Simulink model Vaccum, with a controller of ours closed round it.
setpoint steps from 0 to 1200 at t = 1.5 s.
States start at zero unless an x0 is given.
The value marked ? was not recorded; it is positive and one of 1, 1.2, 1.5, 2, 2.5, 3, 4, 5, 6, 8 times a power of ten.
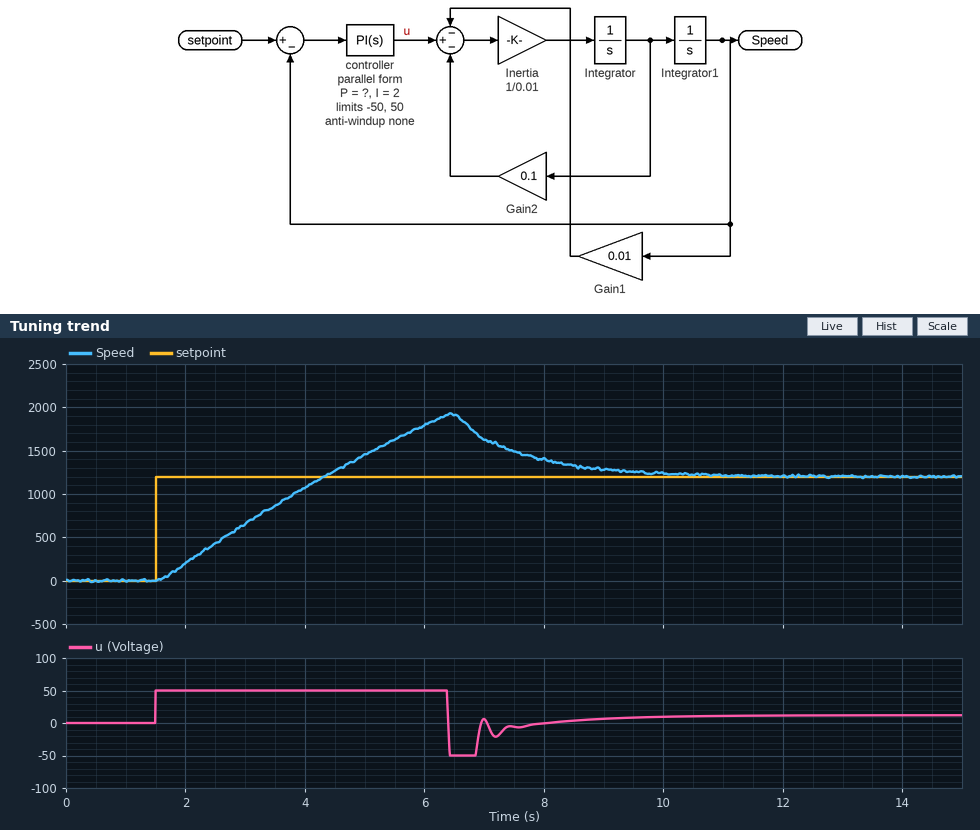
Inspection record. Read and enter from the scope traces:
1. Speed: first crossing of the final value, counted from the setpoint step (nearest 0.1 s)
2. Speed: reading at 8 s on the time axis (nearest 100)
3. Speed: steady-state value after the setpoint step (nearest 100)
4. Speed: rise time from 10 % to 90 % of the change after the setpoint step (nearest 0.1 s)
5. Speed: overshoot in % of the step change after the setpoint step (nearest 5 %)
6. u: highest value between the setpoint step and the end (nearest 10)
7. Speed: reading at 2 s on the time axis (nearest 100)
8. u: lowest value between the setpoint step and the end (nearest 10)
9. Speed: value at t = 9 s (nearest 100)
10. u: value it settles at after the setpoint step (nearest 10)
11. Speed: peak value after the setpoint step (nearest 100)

2.8 s
1400
1200
2.2 s
60 %
50
200
-50
1300
10
1900
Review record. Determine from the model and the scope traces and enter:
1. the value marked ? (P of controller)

2.5
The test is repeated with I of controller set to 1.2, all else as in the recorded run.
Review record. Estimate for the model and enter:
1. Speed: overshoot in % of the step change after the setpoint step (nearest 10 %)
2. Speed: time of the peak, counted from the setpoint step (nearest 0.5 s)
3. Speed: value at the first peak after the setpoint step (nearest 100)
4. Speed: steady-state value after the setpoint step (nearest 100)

50 %
4.5 s
1800
1200
